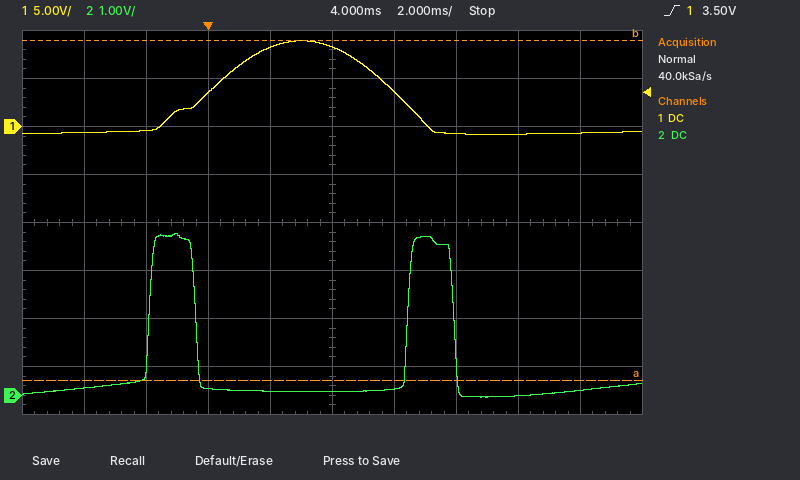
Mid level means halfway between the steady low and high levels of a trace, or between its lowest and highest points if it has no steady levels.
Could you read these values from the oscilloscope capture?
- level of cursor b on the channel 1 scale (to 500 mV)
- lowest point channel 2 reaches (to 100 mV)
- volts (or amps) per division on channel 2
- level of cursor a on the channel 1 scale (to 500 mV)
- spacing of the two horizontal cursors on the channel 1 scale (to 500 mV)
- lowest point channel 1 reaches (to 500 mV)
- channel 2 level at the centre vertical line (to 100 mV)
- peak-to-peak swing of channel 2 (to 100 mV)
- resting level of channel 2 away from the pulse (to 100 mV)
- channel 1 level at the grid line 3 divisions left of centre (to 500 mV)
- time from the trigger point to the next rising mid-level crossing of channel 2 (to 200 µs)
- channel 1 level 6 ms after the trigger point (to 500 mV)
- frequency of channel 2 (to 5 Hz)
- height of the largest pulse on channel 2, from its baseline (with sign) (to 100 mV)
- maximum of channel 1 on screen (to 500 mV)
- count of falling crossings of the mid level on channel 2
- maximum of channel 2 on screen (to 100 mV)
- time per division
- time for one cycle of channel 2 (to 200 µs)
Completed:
9.0 V
0.0 V
1 V
-26.5 V
35.5 V
-1.0 V
100 mV
3.4 V
100 mV
-500 mV
6.4 ms
3.5 V
120 Hz
+3.3 V
9.0 V
2
3.4 V
2 ms
8.4 ms
